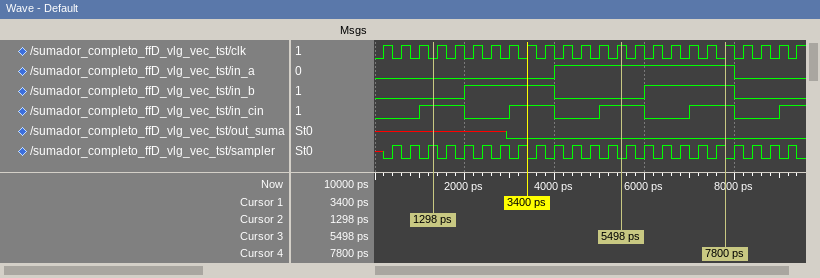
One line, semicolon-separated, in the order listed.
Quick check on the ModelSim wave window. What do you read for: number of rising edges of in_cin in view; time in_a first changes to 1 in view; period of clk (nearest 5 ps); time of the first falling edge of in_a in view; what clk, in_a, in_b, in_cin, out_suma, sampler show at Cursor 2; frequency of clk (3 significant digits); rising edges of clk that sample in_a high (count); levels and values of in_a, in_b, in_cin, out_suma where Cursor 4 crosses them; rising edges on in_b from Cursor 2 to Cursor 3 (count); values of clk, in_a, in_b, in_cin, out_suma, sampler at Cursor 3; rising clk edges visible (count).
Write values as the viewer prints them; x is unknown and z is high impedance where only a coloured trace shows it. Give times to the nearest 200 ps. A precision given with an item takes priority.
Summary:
5; 4000 ps; 400 ps; 8000 ps; clk=0, in_a=0, in_b=0, in_cin=1, out_suma=x, sampler=1; 2.50 GHz; 10; in_a=1, in_b=1, in_cin=1, out_suma=0; 1; clk=1, in_a=1, in_b=0, in_cin=1, out_suma=0, sampler=0; 24
